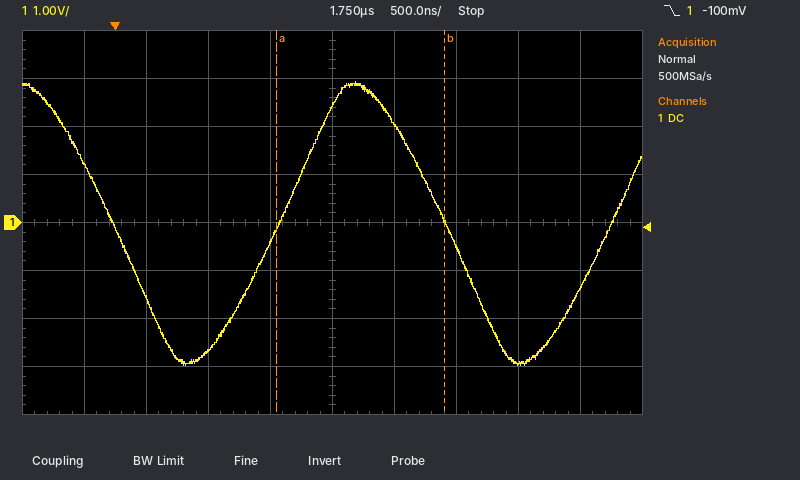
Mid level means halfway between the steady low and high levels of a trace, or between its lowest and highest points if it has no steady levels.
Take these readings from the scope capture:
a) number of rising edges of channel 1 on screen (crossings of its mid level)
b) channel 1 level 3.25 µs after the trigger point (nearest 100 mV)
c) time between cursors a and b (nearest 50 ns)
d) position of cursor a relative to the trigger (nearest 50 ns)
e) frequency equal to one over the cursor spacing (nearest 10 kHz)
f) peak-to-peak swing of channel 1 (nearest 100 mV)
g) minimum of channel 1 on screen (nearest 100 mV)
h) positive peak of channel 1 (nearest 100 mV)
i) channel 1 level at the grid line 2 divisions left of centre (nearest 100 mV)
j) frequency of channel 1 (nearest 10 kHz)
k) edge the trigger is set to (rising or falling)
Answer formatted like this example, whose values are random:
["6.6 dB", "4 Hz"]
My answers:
["2", "-2.9 V", "1.35 µs", "+1.30 µs", "740 kHz", "5.9 V", "-3.0 V", "2.9 V", "-2.7 V", "370 kHz", "falling"]
